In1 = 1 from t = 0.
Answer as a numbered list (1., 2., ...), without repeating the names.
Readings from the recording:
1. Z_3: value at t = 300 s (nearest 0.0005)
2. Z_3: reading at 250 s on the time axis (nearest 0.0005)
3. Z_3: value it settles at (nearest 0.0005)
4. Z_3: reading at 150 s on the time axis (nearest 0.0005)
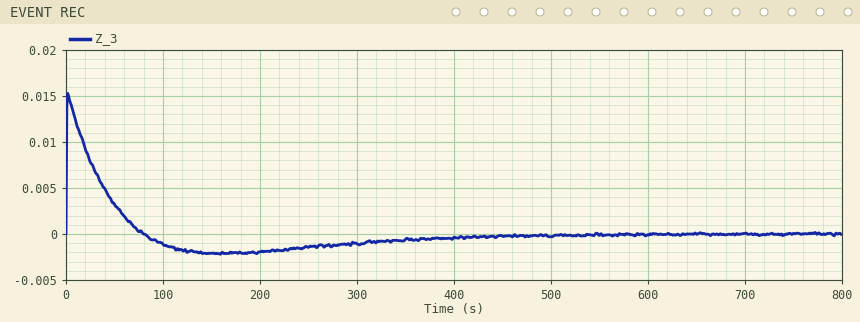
1. -0.0010
2. -0.0015
3. 0.0000
4. -0.0020
